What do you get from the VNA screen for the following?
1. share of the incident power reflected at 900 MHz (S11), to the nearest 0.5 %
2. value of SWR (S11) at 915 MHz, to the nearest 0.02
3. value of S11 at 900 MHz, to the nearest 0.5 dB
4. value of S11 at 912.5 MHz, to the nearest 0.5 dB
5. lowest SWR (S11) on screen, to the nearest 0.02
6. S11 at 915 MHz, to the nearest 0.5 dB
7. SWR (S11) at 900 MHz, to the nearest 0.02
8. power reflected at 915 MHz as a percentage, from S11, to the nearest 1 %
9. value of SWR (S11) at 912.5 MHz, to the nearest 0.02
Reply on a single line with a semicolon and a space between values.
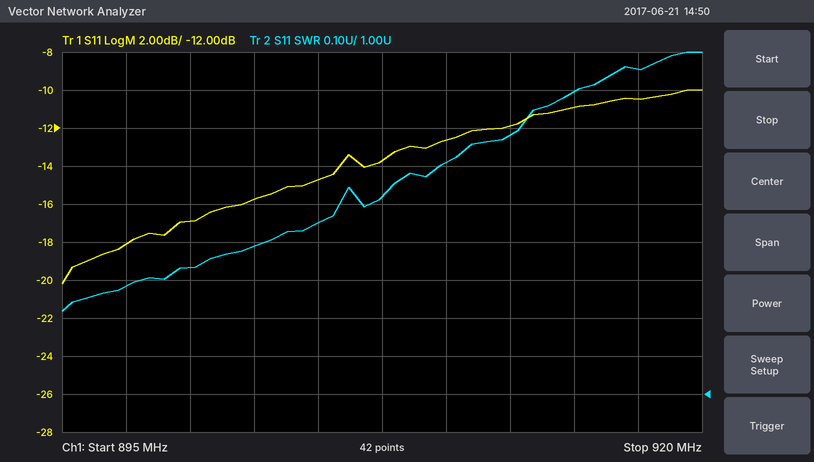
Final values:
2.0 %; 1.80; -17.0 dB; -12.0 dB; 1.22; -11.0 dB; 1.34; 8 %; 1.68
